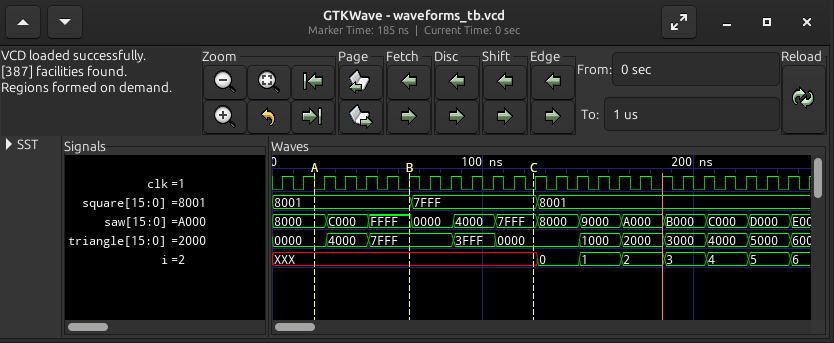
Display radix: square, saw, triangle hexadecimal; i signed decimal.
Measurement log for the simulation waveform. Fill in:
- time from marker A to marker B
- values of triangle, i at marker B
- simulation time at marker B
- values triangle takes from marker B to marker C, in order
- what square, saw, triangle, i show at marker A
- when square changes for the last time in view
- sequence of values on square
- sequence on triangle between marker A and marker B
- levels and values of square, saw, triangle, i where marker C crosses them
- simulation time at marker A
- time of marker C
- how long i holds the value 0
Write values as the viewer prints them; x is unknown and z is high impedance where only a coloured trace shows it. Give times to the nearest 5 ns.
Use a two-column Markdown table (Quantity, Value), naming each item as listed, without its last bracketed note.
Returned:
| Quantity | Value |
|---|---|
| time from marker A to marker B | 45 ns |
| values of triangle, i at marker B | triangle=7FFF, i=XXX |
| simulation time at marker B | 65 ns |
| values triangle takes from marker B to marker C, in order | 7FFF, 3FFF, 0000 |
| what square, saw, triangle, i show at marker A | square=8001, saw=8000, triangle=0000, i=XXX |
| when square changes for the last time in view | 125 ns |
| sequence of values on square | 8001, 7FFF, 8001 |
| sequence on triangle between marker A and marker B | 0000, 4000, 7FFF |
| levels and values of square, saw, triangle, i where marker C crosses them | square=7FFF, saw=7FFF, triangle=0000, i=XXX |
| simulation time at marker A | 20 ns |
| time of marker C | 125 ns |
| how long i holds the value 0 | 20 ns |
